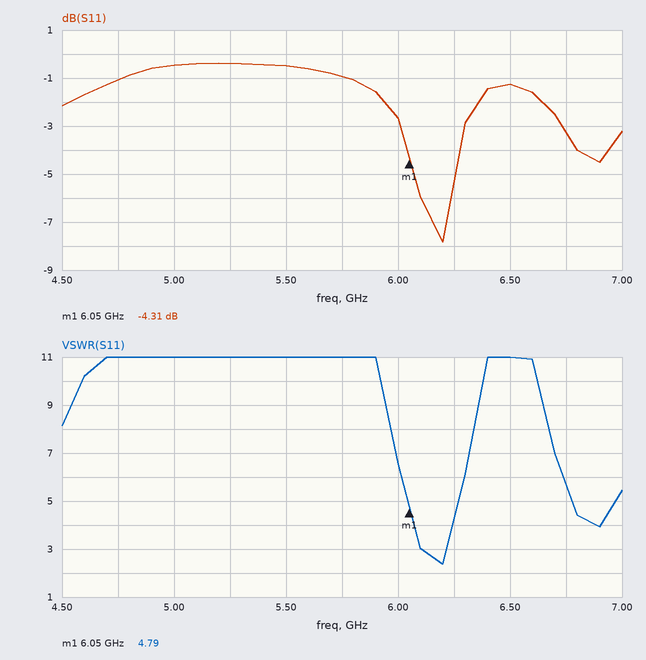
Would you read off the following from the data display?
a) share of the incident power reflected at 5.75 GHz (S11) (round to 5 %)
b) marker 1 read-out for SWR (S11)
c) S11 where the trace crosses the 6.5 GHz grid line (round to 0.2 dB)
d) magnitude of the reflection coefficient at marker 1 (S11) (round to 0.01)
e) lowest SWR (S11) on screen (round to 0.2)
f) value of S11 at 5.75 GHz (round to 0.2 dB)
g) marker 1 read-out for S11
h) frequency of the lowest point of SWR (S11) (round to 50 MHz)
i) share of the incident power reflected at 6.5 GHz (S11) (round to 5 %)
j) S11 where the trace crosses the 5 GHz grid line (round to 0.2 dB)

80 %
4.79
-1.2 dB
0.61
2.4
-1.0 dB
-4.31 dB
6.20 GHz
75 %
-0.4 dB
